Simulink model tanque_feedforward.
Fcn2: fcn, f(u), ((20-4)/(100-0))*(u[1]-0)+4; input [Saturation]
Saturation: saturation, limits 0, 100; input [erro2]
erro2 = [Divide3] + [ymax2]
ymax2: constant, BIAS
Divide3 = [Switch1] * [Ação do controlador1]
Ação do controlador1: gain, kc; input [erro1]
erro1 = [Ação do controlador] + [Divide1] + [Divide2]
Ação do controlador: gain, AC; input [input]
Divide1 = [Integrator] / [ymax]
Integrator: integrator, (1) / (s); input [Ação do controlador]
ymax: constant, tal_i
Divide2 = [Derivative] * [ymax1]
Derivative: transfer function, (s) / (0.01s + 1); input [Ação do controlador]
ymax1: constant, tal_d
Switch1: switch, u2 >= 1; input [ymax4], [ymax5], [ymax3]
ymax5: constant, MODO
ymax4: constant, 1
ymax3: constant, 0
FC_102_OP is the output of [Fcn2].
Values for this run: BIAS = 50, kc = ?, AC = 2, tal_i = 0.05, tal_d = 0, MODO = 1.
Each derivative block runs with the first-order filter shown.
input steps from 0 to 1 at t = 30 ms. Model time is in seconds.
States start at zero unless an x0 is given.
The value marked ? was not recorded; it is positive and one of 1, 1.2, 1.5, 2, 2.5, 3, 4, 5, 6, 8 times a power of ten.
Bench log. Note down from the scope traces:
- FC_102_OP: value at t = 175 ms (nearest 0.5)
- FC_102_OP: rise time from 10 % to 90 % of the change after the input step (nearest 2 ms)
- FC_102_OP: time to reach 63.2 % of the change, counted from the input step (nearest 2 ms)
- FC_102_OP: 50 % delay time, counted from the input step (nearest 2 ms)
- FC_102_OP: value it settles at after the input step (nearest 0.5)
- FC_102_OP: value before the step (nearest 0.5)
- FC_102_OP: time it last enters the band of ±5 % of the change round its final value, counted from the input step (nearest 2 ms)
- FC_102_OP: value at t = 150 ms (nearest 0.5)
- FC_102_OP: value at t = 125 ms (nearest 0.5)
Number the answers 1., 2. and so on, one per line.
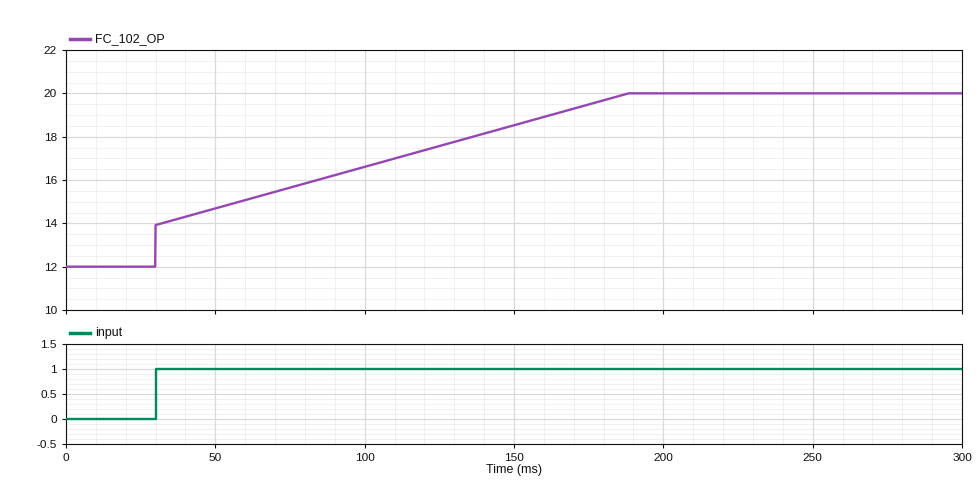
1. 19.5
2. 138 ms
3. 82 ms
4. 54 ms
5. 20.0
6. 12.0
7. 148 ms
8. 18.5
9. 17.5
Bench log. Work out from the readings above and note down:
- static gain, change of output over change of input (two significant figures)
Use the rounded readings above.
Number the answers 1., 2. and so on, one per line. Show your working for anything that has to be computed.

1. (20 - 12) / (1 - 0) = 8.0
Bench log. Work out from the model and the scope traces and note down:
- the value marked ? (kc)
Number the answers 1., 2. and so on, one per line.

1. 6
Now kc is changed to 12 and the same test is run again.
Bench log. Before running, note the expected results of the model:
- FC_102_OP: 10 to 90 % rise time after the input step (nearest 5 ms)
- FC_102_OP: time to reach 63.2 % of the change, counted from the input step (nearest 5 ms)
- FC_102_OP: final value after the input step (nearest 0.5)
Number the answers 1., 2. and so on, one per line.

1. 45 ms
2. 15 ms
3. 20.0
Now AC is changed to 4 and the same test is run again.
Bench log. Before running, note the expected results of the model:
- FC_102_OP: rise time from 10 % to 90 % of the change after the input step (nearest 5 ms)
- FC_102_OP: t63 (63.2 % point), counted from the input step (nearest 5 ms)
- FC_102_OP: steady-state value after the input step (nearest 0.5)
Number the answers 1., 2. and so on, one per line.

1. 45 ms
2. 15 ms
3. 20.0
